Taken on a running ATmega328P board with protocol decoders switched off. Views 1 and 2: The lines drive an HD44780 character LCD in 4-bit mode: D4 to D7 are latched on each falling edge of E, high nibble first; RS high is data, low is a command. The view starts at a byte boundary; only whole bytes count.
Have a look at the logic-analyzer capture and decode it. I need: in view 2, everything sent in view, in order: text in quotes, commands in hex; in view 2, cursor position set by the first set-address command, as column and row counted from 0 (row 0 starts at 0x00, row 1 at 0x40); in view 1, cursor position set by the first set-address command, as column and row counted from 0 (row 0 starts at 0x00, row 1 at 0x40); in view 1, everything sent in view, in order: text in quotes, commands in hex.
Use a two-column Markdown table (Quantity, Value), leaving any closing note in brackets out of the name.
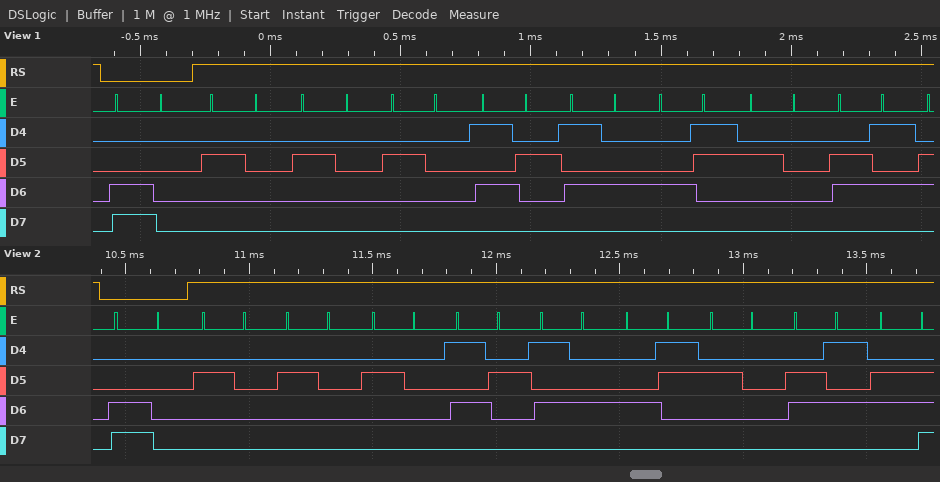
| Quantity | Value |
|---|---|
| in view 2, everything sent in view, in order: text in quotes, commands in hex | 0xC0 "   RTC en" |
| in view 2, cursor position set by the first set-address command, as column and row counted from 0 | column 0, row 1 |
| in view 1, cursor position set by the first set-address command, as column and row counted from 0 | column 0, row 1 |
| in view 1, everything sent in view, in order: text in quotes, commands in hex | 0xC0 "   RTC e" |
